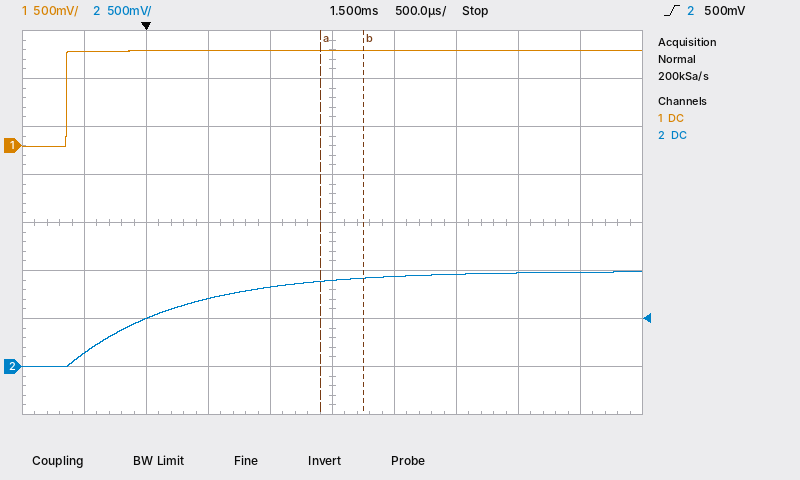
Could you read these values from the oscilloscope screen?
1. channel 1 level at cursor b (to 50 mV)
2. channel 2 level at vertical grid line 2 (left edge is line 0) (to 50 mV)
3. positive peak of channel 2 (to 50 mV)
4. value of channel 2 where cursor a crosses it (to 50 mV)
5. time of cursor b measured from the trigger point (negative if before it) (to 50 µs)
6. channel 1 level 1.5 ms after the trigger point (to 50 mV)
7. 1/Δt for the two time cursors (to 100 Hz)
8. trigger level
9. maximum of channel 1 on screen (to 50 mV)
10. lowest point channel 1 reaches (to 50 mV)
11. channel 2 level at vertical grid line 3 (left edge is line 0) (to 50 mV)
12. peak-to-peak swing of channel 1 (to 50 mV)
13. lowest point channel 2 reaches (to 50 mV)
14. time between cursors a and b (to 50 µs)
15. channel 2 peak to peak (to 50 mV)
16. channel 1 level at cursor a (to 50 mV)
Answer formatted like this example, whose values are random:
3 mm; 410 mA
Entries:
1.00 V; 500 mV; 1.00 V; 900 mV; +1.75 ms; 1.00 V; 2.9 kHz; 500 mV; 1.00 V; 0 mV; 700 mV; 1.00 V; 0 mV; 350 µs; 1.00 V; 1.00 V
